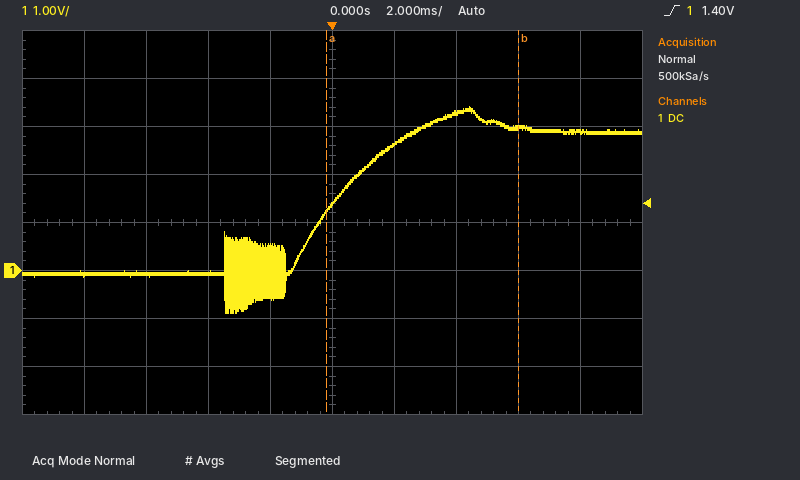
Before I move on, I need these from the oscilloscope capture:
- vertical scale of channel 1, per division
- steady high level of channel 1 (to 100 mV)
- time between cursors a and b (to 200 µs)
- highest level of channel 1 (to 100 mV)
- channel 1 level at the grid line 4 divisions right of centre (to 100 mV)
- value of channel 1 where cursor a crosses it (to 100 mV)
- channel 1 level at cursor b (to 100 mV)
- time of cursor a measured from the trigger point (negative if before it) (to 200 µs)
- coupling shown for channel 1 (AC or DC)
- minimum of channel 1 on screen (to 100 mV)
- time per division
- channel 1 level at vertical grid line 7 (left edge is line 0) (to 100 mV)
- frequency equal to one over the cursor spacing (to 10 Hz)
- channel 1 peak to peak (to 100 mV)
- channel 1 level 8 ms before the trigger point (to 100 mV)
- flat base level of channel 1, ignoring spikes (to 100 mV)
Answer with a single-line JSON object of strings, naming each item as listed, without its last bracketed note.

{"vertical scale of channel 1, per division": "1 V", "steady high level of channel 1": "2.9 V", "time between cursors a and b": "6.2 ms", "highest level of channel 1": "3.4 V", "channel 1 level at the grid line 4 divisions right of centre": "2.9 V", "value of channel 1 where cursor a crosses it": "1.2 V", "channel 1 level at cursor b": "3.0 V", "time of cursor a measured from the trigger point (negative if before it)": "-200 µs", "coupling shown for channel 1": "DC", "minimum of channel 1 on screen": "-900 mV", "time per division": "2 ms", "channel 1 level at vertical grid line 7 (left edge is line 0)": "3.3 V", "frequency equal to one over the cursor spacing": "160 Hz", "channel 1 peak to peak": "4.3 V", "channel 1 level 8 ms before the trigger point": "-100 mV", "flat base level of channel 1, ignoring spikes": "-100 mV"}
